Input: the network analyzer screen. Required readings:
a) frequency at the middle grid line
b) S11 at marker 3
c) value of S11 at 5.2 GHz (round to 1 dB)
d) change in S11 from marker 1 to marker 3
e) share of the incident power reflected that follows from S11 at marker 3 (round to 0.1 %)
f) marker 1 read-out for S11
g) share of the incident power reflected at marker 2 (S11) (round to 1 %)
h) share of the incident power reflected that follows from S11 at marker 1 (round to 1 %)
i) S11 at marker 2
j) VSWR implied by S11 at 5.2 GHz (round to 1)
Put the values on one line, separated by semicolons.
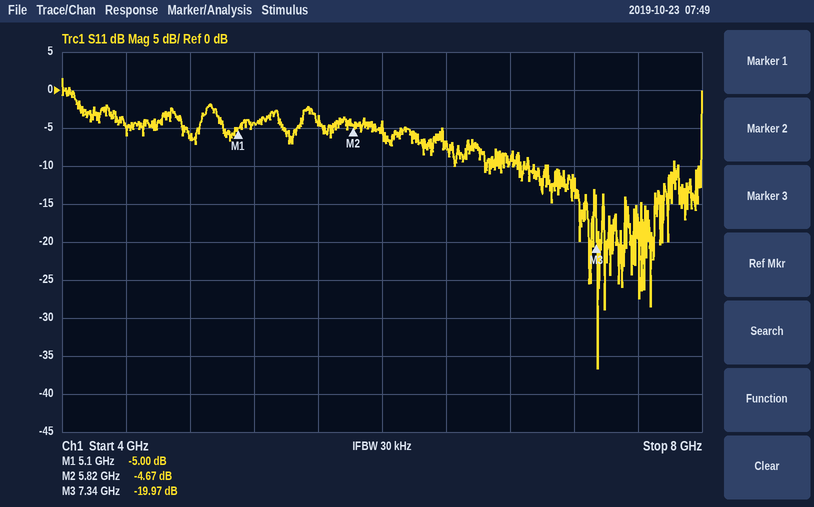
6 GHz; -19.97 dB; -4 dB; -14.97 dB; 1.0 %; -5.00 dB; 34 %; 32 %; -4.67 dB; 4
